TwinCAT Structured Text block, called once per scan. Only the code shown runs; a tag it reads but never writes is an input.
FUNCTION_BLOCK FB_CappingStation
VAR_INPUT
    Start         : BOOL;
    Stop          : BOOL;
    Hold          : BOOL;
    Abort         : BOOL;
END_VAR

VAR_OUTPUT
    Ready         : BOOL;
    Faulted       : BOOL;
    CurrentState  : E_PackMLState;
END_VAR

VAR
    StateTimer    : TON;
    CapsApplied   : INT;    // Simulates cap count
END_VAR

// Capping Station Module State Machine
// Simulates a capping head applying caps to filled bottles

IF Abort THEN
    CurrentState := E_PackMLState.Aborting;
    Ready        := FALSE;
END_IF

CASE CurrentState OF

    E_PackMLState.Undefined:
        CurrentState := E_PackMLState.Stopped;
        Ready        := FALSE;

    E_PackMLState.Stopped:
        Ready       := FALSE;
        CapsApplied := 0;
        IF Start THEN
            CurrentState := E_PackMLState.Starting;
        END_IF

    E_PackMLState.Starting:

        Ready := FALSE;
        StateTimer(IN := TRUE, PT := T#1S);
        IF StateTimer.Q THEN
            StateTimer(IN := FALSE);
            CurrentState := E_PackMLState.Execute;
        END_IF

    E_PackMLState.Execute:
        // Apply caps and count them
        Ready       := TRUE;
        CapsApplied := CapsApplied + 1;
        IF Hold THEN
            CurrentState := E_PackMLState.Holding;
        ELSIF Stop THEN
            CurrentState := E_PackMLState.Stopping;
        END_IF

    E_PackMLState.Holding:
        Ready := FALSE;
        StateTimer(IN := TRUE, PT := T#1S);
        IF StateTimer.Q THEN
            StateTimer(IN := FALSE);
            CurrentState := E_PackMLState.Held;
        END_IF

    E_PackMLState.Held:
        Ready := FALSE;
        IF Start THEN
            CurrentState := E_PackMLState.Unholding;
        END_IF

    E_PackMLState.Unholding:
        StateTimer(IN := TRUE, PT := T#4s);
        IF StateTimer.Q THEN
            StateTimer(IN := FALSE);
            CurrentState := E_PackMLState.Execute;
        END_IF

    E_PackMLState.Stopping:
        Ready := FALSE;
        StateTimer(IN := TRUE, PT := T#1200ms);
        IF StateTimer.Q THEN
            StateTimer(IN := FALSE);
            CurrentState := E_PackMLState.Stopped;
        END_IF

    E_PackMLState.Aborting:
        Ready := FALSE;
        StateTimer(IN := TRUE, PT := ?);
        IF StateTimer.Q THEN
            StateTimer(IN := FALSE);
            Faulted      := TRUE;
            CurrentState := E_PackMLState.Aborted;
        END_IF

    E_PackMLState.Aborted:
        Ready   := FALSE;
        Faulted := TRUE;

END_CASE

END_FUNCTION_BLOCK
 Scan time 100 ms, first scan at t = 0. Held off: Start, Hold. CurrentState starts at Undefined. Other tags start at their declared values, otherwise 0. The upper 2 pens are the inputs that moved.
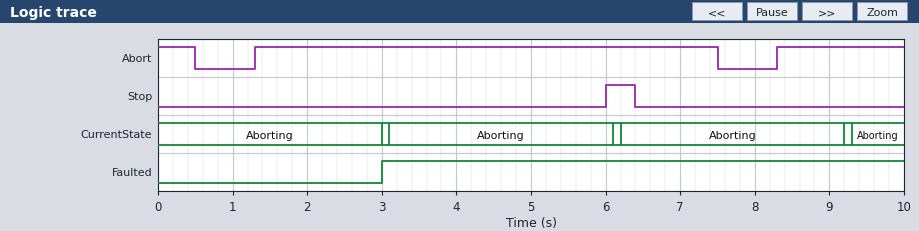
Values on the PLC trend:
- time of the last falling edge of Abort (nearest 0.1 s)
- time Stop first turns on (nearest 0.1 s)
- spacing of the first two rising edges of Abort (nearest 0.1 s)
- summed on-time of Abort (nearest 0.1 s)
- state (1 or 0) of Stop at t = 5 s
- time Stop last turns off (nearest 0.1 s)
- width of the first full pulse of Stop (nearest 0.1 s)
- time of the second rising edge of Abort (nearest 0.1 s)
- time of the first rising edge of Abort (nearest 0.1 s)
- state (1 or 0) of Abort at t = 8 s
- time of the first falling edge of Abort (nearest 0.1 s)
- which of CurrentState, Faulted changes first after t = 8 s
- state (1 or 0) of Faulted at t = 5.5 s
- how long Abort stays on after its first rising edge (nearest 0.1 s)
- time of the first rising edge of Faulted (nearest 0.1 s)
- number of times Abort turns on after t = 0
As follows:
7.5 s
6.0 s
7.0 s
8.4 s
0
6.4 s
0.4 s
8.3 s
1.3 s
0
0.5 s
CurrentState
1
6.2 s
3.0 s
2
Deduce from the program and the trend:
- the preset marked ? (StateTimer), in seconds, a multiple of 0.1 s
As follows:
3.0 s
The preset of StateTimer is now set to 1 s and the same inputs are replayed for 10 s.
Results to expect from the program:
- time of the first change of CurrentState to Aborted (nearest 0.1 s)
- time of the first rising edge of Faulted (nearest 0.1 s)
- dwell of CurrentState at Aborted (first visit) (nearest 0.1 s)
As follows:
1.0 s
1.0 s
0.3 s
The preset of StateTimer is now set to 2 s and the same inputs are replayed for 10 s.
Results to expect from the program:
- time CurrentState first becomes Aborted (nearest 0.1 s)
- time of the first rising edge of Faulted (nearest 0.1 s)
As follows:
2.0 s
2.0 s
